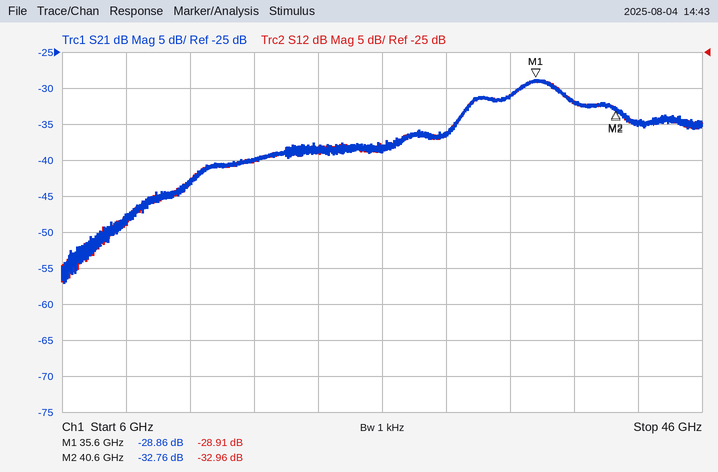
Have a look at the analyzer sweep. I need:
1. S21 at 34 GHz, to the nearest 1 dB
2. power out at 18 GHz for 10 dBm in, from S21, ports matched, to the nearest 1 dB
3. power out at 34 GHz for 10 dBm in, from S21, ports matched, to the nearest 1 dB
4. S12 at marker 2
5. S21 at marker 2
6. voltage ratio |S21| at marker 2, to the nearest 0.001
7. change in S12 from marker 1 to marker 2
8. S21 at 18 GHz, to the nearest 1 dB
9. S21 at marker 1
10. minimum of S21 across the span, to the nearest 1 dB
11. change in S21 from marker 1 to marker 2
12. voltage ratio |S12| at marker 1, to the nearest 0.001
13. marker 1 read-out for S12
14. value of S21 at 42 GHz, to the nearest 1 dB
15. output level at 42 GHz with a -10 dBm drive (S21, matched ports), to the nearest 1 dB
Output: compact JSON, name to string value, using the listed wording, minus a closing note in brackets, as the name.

{"S21 at 34 GHz, to the nearest 1 dB": "-31 dB", "power out at 18 GHz for 10 dBm in, from S21, ports matched, to the nearest 1 dB": "-30 dBm", "power out at 34 GHz for 10 dBm in, from S21, ports matched, to the nearest 1 dB": "-21 dBm", "S12 at marker 2": "-32.96 dB", "S21 at marker 2": "-32.76 dB", "voltage ratio |S21| at marker 2, to the nearest 0.001": "0.023", "change in S12 from marker 1 to marker 2": "-4.05 dB", "S21 at 18 GHz, to the nearest 1 dB": "-40 dB", "S21 at marker 1": "-28.86 dB", "minimum of S21 across the span, to the nearest 1 dB": "-57 dB", "change in S21 from marker 1 to marker 2": "-3.90 dB", "voltage ratio |S12| at marker 1, to the nearest 0.001": "0.036", "marker 1 read-out for S12": "-28.91 dB", "value of S21 at 42 GHz, to the nearest 1 dB": "-35 dB", "output level at 42 GHz with a -10 dBm drive (S21, matched ports), to the nearest 1 dB": "-45 dBm"}
